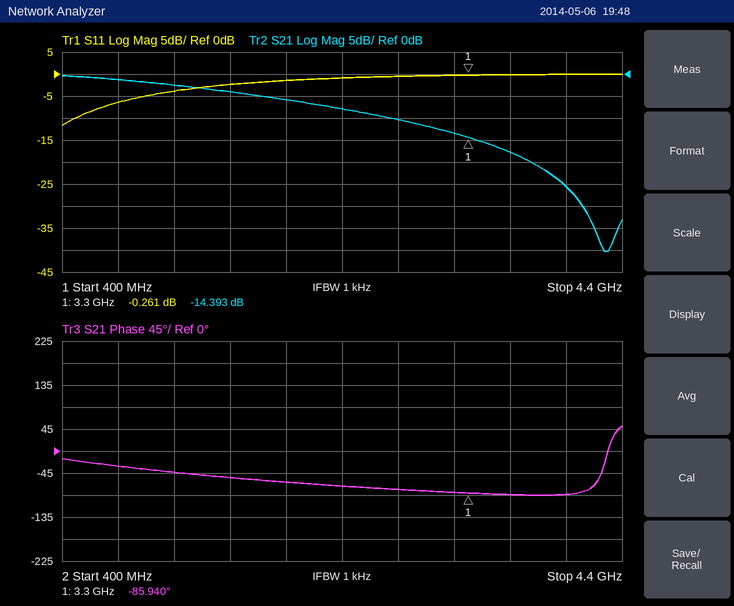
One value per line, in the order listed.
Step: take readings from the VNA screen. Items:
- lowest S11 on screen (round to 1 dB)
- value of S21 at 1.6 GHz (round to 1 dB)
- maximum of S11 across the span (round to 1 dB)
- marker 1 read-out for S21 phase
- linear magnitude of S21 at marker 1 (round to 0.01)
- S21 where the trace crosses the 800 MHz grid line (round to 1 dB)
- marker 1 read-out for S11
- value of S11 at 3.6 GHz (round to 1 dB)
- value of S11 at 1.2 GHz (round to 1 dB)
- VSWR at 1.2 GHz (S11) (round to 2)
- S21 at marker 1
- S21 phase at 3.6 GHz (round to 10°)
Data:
-12 dB
-4 dB
0 dB
-85.940°
0.19
-1 dB
-0.261 dB
0 dB
-4 dB
4
-14.393 dB
-90°
